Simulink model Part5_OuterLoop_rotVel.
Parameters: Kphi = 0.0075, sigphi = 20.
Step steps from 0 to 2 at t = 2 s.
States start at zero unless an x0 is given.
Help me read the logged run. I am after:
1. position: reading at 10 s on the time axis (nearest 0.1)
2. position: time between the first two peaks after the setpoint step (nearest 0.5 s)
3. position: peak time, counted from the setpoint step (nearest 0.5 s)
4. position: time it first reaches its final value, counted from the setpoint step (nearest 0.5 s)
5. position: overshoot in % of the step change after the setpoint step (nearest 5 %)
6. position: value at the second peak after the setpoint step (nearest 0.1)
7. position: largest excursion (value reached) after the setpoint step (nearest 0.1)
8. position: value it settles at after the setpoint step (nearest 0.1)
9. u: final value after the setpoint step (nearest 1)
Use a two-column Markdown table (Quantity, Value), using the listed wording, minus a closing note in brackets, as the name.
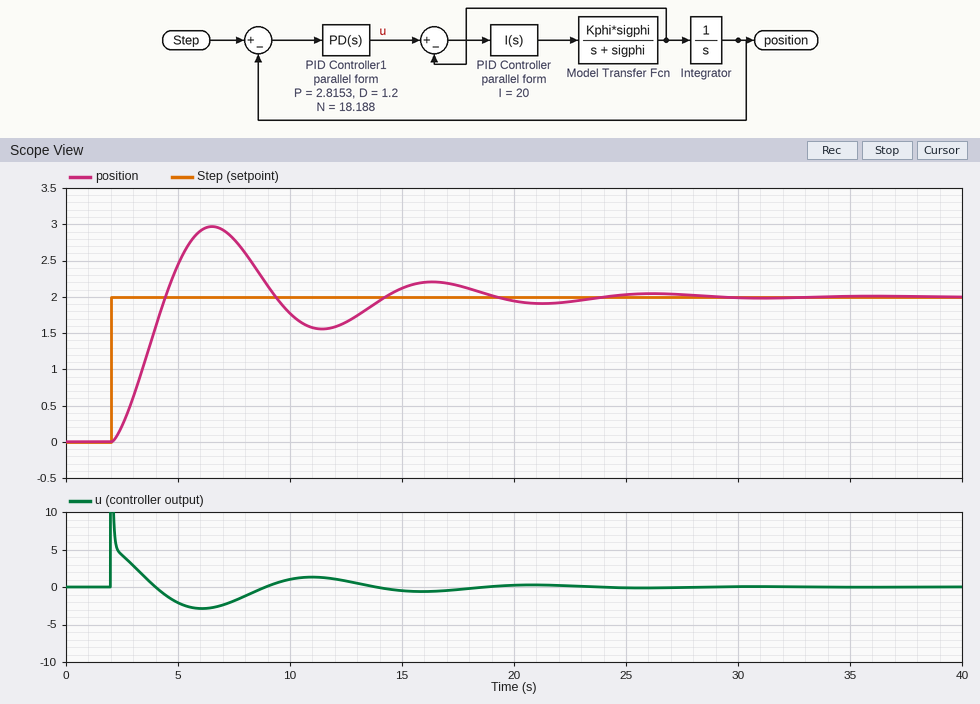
| Quantity | Value |
|---|---|
| position: reading at 10 s on the time axis | 1.8 |
| position: time between the first two peaks after the setpoint step | 10.0 s |
| position: peak time, counted from the setpoint step | 4.5 s |
| position: time it first reaches its final value, counted from the setpoint step | 2.5 s |
| position: overshoot in % of the step change after the setpoint step | 50 % |
| position: value at the second peak after the setpoint step | 2.2 |
| position: largest excursion (value reached) after the setpoint step | 3.0 |
| position: value it settles at after the setpoint step | 2.0 |
| u: final value after the setpoint step | 0 |
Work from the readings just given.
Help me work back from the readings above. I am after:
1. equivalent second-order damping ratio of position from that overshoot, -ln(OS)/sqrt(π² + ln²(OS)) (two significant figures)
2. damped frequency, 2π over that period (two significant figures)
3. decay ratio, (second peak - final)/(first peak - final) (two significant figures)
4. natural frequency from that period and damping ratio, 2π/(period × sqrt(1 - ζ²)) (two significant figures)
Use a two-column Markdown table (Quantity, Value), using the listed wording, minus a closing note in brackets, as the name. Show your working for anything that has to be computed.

| Quantity | Value |
|---|---|
| equivalent second-order damping ratio of position from that overshoot, -ln(OS)/sqrt(π² + ln²(OS)) | ln(0.5) = -0.693; 0.693 / sqrt(9.870 + 0.480) = 0.22 |
| damped frequency, 2π over that period | 2π / 10 = 0.63 rad/s |
| decay ratio, (second peak - final)/(first peak - final) | (2.2 - 2) / (3 - 2) = 0.20 |
| natural frequency from that period and damping ratio, 2π/(period × sqrt(1 - ζ²)) | 2π / (10 × sqrt(1 - 0.22²)) = 0.64 rad/s |
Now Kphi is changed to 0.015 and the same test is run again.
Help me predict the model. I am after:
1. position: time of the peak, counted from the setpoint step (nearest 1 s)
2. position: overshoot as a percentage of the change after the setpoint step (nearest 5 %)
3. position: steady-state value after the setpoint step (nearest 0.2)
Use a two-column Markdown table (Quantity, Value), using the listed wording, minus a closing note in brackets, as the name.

| Quantity | Value |
|---|---|
| position: time of the peak, counted from the setpoint step | 3 s |
| position: overshoot as a percentage of the change after the setpoint step | 35 % |
| position: steady-state value after the setpoint step | 2.0 |
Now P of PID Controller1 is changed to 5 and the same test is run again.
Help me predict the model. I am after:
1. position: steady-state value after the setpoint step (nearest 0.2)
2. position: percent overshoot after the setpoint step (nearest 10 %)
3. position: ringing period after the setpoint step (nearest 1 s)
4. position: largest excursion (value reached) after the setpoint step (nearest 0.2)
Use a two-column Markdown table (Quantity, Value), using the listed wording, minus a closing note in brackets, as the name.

| Quantity | Value |
|---|---|
| position: steady-state value after the setpoint step | 2.0 |
| position: percent overshoot after the setpoint step | 60 % |
| position: ringing period after the setpoint step | 7 s |
| position: largest excursion (value reached) after the setpoint step | 3.2 |
